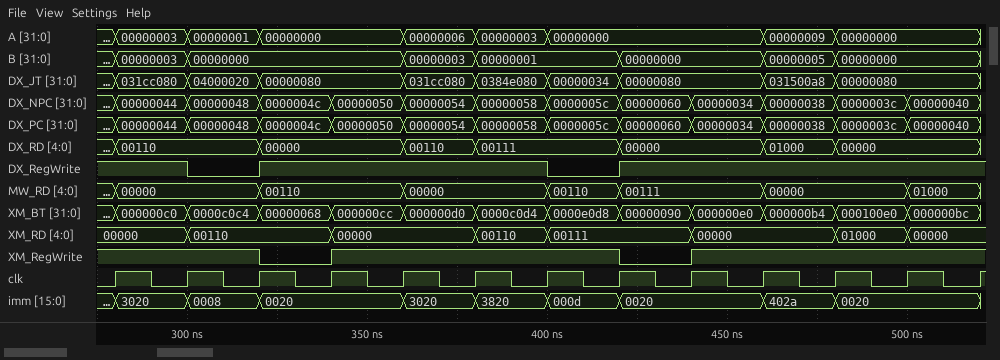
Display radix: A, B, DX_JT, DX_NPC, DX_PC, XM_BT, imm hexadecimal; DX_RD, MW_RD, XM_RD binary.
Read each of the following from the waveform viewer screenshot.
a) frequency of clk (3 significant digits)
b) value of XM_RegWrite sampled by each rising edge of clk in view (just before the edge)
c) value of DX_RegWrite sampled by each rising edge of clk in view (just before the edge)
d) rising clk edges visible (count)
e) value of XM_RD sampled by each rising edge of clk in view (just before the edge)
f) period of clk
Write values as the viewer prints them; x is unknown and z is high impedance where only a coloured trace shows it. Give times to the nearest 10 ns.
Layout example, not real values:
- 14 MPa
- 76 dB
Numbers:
- 50.0 MHz
- 1 1 1 0 1 1 1 1 0 1 1 1 1
- 1 1 0 1 1 1 1 0 1 1 1 1 1
- 13
- 00000, 00000, 00110, 00110, 00000, 00000, 00110, 00111, 00111, 00000, 00000, 01000, 00000
- 20 ns
